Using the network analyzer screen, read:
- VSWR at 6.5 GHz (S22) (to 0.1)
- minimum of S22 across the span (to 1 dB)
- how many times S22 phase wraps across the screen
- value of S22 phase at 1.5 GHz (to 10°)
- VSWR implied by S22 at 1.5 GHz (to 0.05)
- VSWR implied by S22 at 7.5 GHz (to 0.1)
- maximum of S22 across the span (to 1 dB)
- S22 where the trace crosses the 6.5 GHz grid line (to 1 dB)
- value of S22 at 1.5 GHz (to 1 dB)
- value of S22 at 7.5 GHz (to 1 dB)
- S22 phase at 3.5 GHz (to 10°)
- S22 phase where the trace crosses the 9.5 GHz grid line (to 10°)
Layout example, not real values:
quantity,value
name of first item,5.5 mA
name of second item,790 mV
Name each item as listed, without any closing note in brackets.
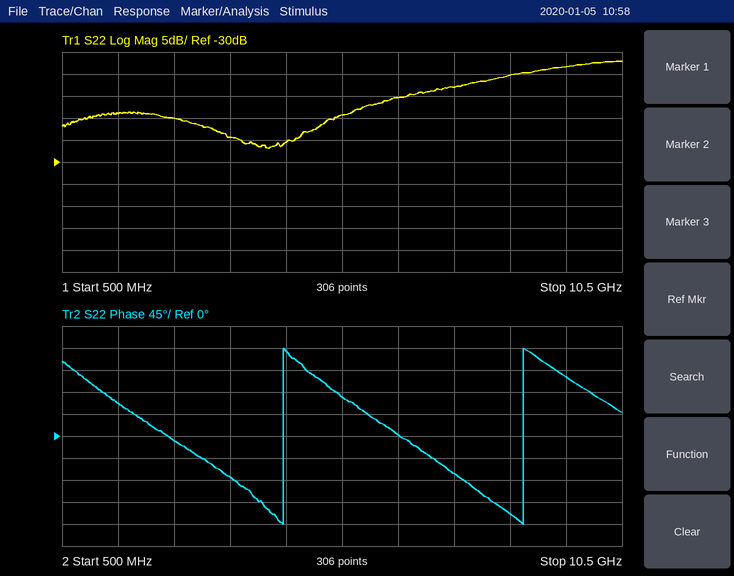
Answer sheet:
quantity,value
VSWR at 6.5 GHz (S22),1.4
minimum of S22 across the span,-27 dB
how many times S22 phase wraps across the screen,2
value of S22 phase at 1.5 GHz,70°
VSWR implied by S22 at 1.5 GHz,1.25
VSWR implied by S22 at 7.5 GHz,1.6
maximum of S22 across the span,-7 dB
S22 where the trace crosses the 6.5 GHz grid line,-15 dB
value of S22 at 1.5 GHz,-19 dB
value of S22 at 7.5 GHz,-13 dB
S22 phase at 3.5 GHz,-80°
S22 phase where the trace crosses the 9.5 GHz grid line,120°
